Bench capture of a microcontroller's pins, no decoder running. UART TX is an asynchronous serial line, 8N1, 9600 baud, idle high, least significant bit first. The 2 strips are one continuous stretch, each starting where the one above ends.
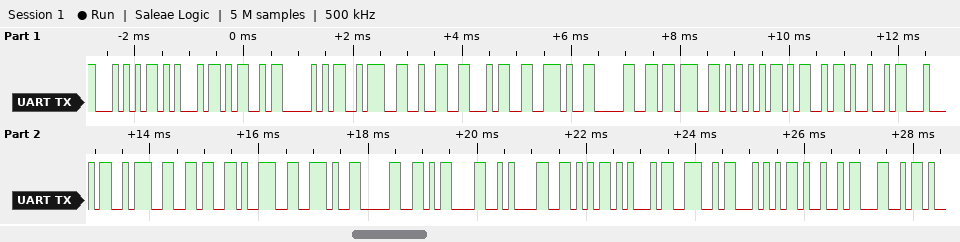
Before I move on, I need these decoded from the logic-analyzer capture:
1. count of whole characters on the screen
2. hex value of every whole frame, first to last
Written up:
27
0x54 0x45 0x4D 0x50 0x3A 0x32 0x34 0x2E 0x30 0x3B 0x55 0x4D 0x49 0x44 0x3A 0x36 0x39 0x2E 0x30 0x0D 0x0A 0x56 0x45 0x4E 0x54 0x49 0x4C
